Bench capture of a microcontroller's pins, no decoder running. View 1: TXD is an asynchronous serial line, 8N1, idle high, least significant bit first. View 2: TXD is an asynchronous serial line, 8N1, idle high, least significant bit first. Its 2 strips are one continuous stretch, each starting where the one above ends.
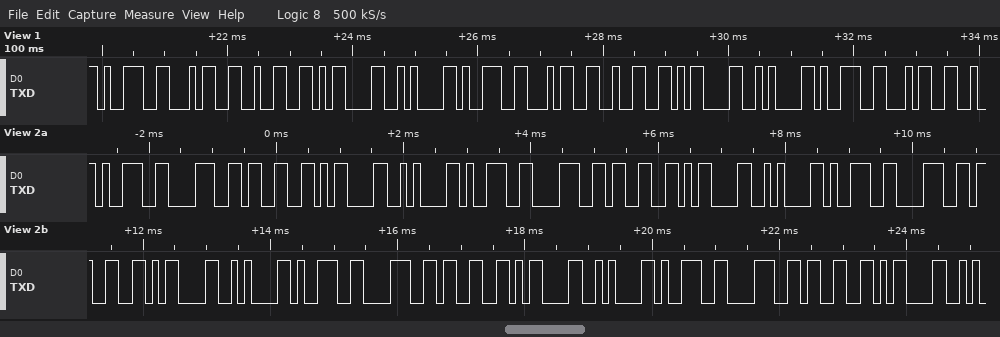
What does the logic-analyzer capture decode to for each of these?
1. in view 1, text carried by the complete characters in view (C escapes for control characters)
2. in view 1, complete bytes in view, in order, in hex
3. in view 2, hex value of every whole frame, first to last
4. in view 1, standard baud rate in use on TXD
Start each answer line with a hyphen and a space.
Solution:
- "942\r\n942\r\n94"
- 39 34 32 0D 0A 39 34 32 0D 0A 39 34
- 39 38 33 0D 0A 39 38 33 0D 0A 39 38 33 0D 0A 39 38 33 0D 0A 39 38 33 0D
- 9600 baud
